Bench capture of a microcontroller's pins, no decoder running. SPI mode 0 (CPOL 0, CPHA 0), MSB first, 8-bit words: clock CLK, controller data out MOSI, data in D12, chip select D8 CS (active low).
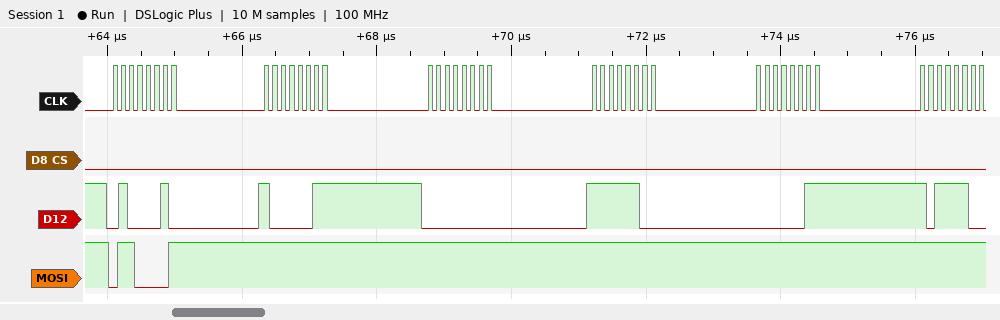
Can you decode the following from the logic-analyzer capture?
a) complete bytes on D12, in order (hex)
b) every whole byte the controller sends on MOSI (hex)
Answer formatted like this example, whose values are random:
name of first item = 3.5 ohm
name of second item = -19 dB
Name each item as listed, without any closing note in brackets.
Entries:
complete bytes on D12, in order = 42 83 00 FC 03 BC
every whole byte the controller sends on MOSI = 61 FF FF FF FF FF
